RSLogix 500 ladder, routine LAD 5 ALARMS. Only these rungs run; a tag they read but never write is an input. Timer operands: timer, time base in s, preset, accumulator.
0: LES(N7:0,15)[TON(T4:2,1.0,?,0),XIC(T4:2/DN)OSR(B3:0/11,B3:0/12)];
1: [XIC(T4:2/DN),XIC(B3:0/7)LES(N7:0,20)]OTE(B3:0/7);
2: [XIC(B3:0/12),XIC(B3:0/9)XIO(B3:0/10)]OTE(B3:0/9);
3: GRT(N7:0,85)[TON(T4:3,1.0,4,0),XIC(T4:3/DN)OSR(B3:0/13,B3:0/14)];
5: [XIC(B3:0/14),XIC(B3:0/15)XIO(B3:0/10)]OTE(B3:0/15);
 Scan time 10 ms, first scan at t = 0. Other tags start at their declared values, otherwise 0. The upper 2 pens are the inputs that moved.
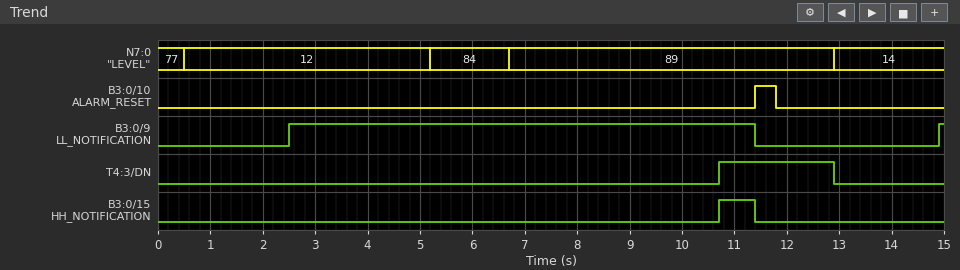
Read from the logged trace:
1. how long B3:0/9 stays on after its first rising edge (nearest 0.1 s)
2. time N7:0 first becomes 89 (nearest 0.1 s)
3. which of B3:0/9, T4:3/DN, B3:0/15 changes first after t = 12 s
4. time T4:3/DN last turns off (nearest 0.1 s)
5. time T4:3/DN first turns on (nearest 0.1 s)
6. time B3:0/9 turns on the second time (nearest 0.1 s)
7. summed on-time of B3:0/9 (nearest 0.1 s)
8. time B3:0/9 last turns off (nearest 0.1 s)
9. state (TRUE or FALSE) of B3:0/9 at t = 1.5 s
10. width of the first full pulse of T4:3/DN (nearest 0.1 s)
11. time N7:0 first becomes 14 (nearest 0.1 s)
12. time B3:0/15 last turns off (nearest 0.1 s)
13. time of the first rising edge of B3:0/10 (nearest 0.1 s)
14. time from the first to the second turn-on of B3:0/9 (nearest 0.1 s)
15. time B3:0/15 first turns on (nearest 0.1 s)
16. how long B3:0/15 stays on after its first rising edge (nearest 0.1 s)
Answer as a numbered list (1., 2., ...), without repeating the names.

1. 8.9 s
2. 6.7 s
3. T4:3/DN
4. 12.9 s
5. 10.7 s
6. 14.9 s
7. 9.0 s
8. 11.4 s
9. FALSE
10. 2.2 s
11. 12.9 s
12. 11.4 s
13. 11.4 s
14. 12.4 s
15. 10.7 s
16. 0.7 s
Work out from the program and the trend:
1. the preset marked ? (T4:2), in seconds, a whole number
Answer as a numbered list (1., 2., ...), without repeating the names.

1. 2 s
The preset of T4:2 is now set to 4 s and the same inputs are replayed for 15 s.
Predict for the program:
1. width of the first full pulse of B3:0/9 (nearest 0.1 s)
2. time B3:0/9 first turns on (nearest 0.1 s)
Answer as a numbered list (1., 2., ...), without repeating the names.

1. 6.9 s
2. 4.5 s
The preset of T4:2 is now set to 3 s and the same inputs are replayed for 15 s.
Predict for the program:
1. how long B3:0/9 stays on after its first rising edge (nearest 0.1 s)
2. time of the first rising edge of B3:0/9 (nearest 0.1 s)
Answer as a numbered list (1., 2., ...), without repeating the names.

1. 7.9 s
2. 3.5 s
